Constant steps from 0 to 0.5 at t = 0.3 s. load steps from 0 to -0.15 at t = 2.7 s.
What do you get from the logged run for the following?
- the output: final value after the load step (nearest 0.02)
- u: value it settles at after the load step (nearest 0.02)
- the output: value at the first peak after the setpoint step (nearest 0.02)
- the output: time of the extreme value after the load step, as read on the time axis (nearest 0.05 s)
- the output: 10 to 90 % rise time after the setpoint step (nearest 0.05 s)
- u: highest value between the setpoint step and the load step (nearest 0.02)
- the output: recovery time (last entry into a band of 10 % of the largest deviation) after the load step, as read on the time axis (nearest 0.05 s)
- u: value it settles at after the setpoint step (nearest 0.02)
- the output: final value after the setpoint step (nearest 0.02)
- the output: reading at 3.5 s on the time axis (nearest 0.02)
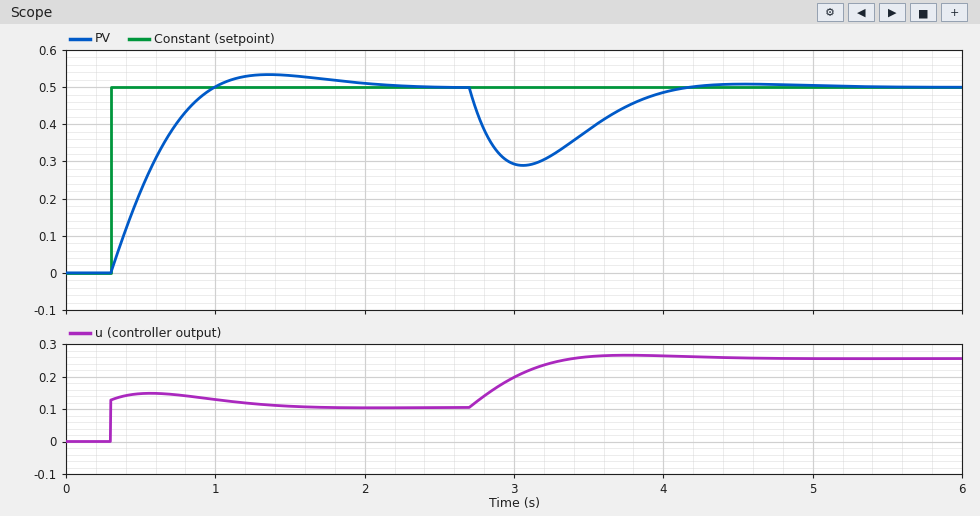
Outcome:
0.50
0.26
0.54
3.05 s
0.50 s
0.14
3.95 s
0.10
0.50
0.38
